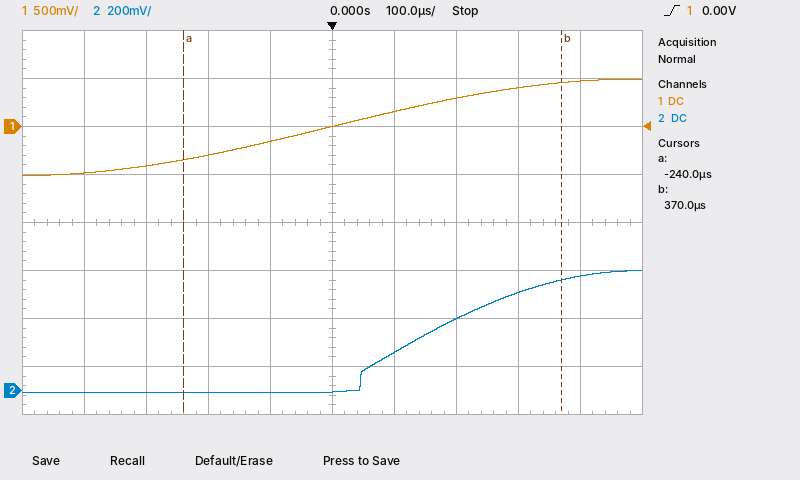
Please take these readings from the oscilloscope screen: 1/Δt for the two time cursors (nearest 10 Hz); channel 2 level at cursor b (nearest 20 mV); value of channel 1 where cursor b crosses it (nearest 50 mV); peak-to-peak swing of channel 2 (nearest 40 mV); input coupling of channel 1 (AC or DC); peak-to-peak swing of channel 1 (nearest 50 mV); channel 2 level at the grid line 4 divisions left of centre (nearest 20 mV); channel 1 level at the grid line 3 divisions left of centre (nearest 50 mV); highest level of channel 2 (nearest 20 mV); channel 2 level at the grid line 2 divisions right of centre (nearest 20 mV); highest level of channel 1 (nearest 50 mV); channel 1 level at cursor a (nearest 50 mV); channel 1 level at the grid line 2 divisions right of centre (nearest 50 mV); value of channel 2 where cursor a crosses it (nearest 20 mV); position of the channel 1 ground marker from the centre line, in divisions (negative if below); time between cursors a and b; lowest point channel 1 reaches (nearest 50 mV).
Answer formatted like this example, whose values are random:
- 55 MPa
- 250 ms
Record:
- 1.64 kHz
- 460 mV
- 450 mV
- 520 mV
- DC
- 1.00 V
- 0 mV
- -400 mV
- 500 mV
- 300 mV
- 500 mV
- -350 mV
- 300 mV
- 0 mV
- +2.0 div
- 610 µs
- -500 mV
